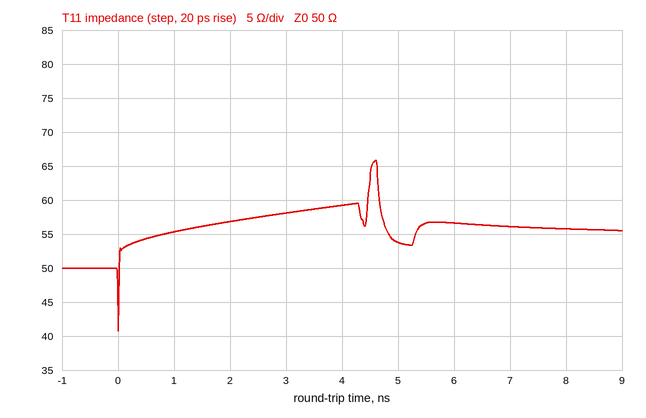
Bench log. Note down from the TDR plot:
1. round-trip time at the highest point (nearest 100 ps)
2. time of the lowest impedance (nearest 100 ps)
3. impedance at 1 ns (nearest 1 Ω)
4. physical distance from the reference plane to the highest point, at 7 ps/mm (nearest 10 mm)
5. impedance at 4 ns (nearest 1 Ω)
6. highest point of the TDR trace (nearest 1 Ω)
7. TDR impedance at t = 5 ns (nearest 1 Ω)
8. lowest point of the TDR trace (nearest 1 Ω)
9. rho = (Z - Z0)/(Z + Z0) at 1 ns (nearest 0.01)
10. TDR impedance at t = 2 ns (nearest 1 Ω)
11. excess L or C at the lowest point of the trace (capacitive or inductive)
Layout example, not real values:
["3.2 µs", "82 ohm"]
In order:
["4.6 ns", "0.0 ns", "55 Ω", "330 mm", "59 Ω", "66 Ω", "54 Ω", "41 Ω", "+0.05", "57 Ω", "capacitive"]
